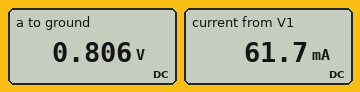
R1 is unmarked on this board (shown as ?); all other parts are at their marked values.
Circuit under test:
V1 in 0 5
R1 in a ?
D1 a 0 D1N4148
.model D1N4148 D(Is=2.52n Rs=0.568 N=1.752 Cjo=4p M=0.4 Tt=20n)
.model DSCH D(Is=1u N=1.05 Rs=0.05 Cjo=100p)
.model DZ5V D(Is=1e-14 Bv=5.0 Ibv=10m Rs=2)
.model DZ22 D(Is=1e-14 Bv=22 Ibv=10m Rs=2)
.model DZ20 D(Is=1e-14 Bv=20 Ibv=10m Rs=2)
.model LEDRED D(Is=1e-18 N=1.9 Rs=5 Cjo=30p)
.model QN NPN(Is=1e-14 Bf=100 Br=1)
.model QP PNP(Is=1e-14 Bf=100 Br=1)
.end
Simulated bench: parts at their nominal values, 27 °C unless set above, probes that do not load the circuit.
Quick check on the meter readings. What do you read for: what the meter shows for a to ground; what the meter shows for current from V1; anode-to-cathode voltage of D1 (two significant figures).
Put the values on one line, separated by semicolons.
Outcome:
0.806 V; 61.7 mA; 810 mV
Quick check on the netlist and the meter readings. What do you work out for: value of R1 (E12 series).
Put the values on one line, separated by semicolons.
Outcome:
68 Ω
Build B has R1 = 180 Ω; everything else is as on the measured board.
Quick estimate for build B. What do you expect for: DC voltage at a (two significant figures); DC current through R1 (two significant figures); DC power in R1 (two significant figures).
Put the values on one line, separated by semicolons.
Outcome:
740 mV; 24 mA; 100 mW
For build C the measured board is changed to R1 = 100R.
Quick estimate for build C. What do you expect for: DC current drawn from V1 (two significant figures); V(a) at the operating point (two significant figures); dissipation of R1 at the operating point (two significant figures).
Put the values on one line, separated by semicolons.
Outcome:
42 mA; 780 mV; 180 mW
